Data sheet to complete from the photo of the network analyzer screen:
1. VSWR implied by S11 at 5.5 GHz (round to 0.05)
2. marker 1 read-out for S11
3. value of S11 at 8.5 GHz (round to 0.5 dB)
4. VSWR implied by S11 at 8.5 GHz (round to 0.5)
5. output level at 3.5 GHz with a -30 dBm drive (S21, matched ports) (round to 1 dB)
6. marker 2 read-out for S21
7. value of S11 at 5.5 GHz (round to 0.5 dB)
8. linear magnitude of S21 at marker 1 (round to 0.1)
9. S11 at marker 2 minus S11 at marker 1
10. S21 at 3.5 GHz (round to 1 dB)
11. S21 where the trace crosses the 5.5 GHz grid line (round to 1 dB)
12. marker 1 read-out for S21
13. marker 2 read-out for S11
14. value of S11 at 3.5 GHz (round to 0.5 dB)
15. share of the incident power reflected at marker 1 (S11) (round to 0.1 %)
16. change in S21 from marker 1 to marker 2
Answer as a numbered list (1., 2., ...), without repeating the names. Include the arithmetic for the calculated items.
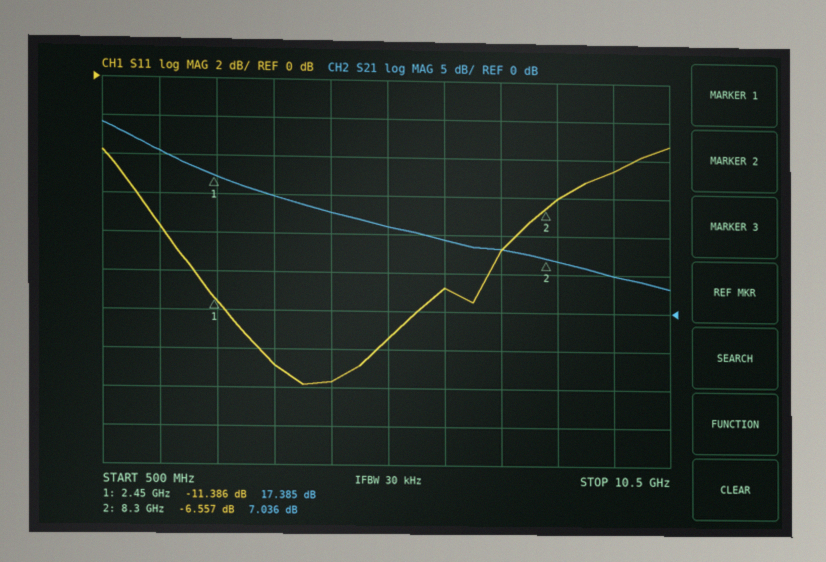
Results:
1. |Γ| = 10^(-13.5/20) = 0.2113; VSWR = (1 + 0.2113)/(1 − 0.2113) ≈ 1.54, so 1.55 to the nearest 0.05
2. -11.386 dB
3. -6.0 dB
4. |Γ| = 10^(-6/20) = 0.5012; VSWR = (1 + 0.5012)/(1 − 0.5012) ≈ 3.0
5. -30 dBm + (15 dB) = -15 dBm
6. 7.036 dB
7. -13.5 dB
8. 10^(17.385/20) ≈ 7.4
9. -6.557 − (-11.386) = 4.829 dB
10. 15 dB
11. 11 dB
12. 17.385 dB
13. -6.557 dB
14. -15.0 dB
15. 10^(-11.386/10) ≈ 7.3 %
16. 7.036 − (17.385) = -10.349 dB
